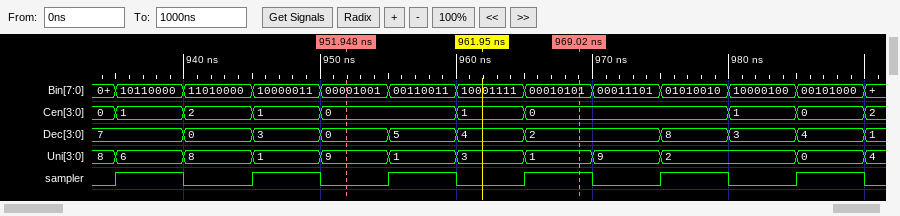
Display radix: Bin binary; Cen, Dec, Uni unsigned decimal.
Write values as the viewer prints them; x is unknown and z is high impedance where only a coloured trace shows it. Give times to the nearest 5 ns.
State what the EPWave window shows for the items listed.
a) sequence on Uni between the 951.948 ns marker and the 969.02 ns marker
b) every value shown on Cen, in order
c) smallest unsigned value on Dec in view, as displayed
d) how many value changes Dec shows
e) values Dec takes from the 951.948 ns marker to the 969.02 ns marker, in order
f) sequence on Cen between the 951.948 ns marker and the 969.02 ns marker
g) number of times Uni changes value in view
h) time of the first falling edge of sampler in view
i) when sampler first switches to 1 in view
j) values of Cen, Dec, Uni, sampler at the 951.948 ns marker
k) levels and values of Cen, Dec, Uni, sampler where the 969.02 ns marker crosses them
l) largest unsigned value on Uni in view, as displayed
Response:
9, 1, 3, 1
0, 1, 2, 1, 0, 1, 0, 1, 0, 2
0
10
0, 5, 4, 2
0, 1, 0
11
940 ns
935 ns
Cen=0, Dec=0, Uni=9, sampler=0
Cen=0, Dec=2, Uni=1, sampler=1
9
